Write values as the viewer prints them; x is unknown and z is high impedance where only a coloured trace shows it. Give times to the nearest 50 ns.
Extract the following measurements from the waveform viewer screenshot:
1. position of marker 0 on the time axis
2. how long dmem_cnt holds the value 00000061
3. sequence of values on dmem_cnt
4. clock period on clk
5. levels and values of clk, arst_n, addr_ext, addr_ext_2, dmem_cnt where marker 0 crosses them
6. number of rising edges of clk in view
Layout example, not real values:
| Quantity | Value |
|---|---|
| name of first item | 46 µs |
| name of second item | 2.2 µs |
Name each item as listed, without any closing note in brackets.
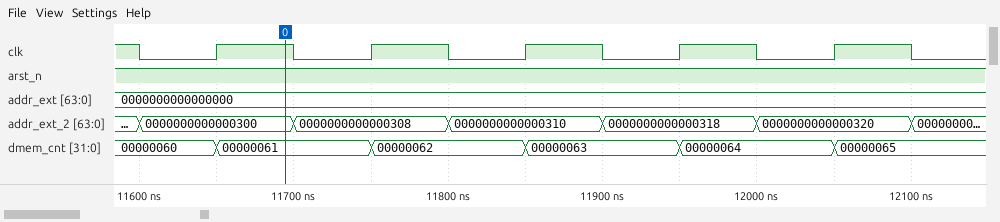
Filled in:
| Quantity | Value |
|---|---|
| position of marker 0 on the time axis | 11700 ns |
| how long dmem_cnt holds the value 00000061 | 100 ns |
| sequence of values on dmem_cnt | 00000060, 00000061, 00000062, 00000063, 00000064, 00000065 |
| clock period on clk | 100 ns |
| levels and values of clk, arst_n, addr_ext, addr_ext_2, dmem_cnt where marker 0 crosses them | clk=1, arst_n=1, addr_ext=0000000000000000, addr_ext_2=0000000000000300, dmem_cnt=00000061 |
| number of rising edges of clk in view | 5 |
